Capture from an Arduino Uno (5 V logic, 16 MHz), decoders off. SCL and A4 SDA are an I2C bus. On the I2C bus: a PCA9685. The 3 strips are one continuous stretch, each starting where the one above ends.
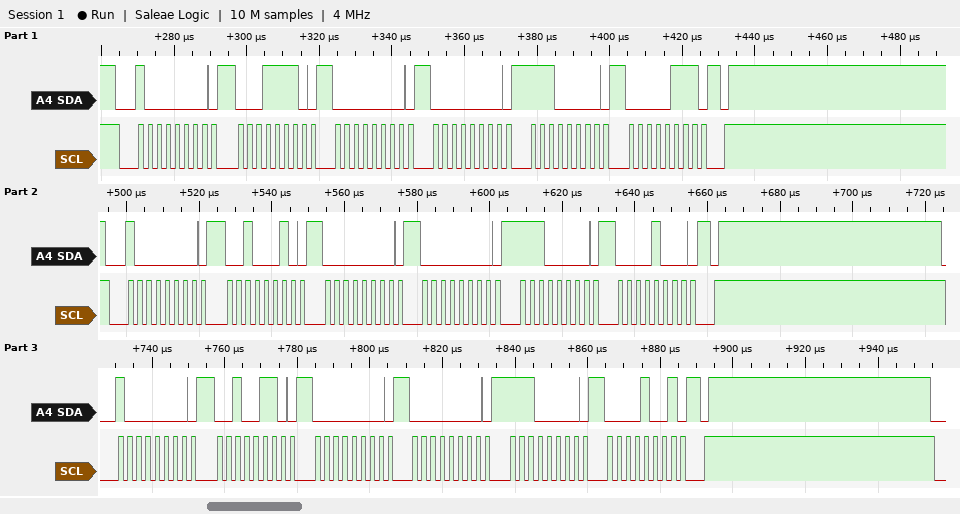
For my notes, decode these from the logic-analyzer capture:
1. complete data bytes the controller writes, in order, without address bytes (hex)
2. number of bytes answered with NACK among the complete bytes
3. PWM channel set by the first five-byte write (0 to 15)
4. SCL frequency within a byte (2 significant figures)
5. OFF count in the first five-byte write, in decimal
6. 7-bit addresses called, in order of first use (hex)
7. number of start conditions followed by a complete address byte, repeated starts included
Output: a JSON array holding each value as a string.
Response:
["1E 00 00 E0 07 22 00 00 E0 08 26 00 00 E0 09", "0", "6", "400 kHz", "2016", "0x40", "3"]
